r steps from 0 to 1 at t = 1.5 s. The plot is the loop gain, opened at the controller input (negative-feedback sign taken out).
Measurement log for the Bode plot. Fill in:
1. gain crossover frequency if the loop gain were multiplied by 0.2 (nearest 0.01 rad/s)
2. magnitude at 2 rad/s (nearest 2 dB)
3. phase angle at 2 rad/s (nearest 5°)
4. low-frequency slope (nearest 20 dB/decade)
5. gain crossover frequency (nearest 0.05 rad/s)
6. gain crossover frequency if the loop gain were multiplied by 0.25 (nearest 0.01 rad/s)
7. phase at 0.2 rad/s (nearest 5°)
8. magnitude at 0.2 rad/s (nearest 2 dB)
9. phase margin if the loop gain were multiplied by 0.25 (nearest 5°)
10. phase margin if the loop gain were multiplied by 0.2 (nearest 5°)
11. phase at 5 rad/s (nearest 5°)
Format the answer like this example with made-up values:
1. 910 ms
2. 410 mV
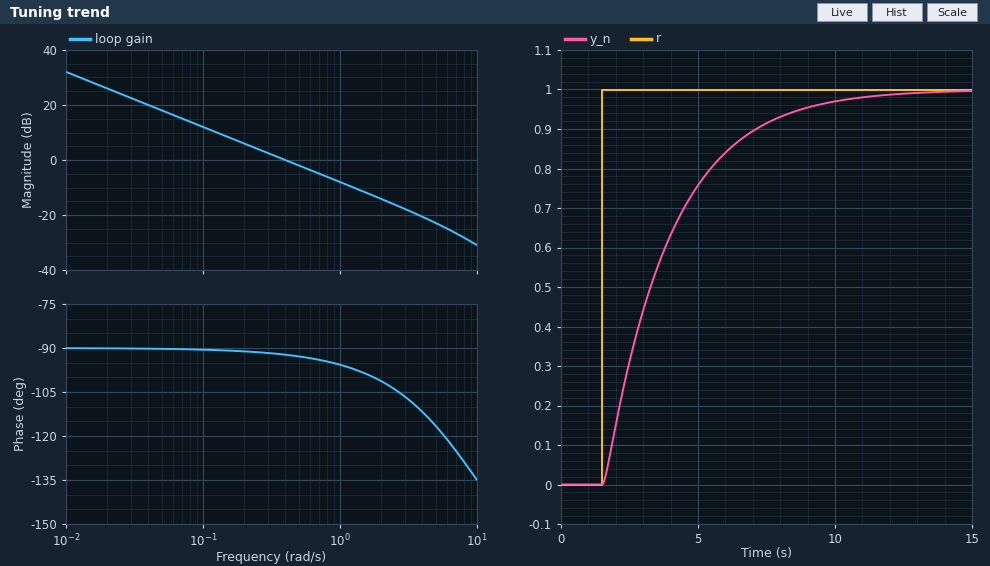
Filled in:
1. 0.08 rad/s
2. -14 dB
3. -100°
4. -20 dB/decade
5. 0.40 rad/s
6. 0.10 rad/s
7. -90°
8. 6 dB
9. 90°
10. 90°
11. -115°
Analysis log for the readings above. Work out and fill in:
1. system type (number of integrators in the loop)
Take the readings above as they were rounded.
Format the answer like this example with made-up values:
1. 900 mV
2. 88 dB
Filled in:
1. 1
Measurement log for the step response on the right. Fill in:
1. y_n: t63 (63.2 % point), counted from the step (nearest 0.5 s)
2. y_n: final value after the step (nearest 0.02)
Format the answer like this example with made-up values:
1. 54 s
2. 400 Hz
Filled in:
1. 2.5 s
2. 1.00
